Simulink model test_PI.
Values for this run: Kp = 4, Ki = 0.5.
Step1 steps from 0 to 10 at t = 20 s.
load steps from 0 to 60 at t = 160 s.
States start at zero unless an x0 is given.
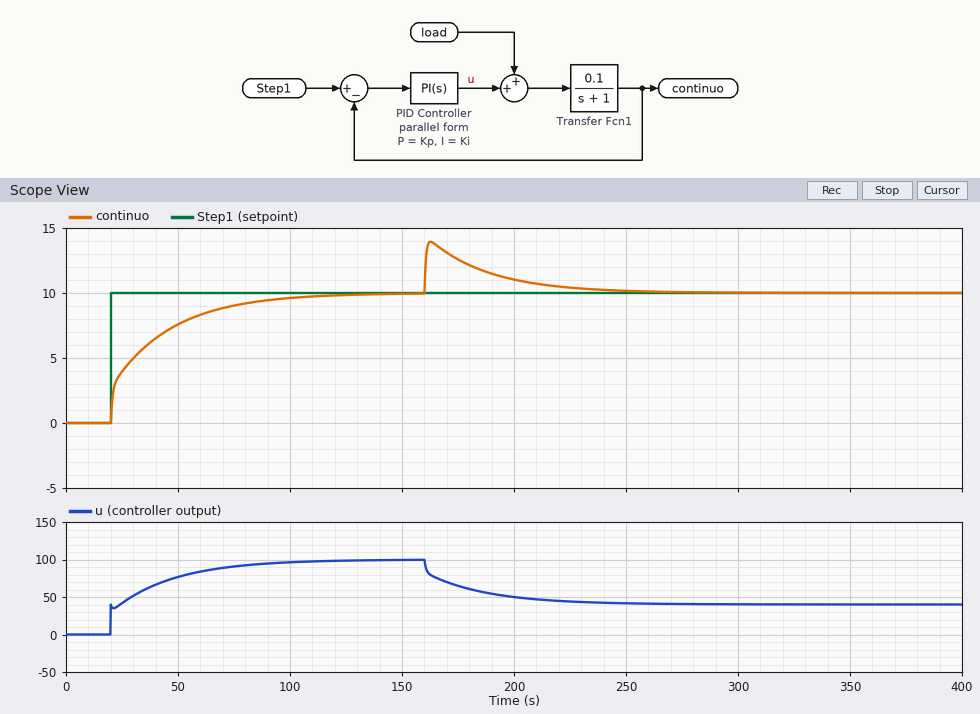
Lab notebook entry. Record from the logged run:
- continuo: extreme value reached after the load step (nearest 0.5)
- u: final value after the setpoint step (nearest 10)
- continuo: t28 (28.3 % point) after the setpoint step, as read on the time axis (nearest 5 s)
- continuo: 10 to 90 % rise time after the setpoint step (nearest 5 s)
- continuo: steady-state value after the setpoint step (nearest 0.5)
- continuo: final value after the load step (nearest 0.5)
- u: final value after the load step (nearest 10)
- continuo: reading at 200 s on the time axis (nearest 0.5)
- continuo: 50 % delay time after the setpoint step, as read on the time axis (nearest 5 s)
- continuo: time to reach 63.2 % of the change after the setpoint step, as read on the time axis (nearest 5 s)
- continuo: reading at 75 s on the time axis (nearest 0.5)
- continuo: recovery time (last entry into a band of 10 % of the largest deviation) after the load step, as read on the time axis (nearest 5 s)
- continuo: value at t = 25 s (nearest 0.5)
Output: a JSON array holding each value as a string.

["14.0", "100", "20 s", "55 s", "10.0", "10.0", "40", "11.0", "30 s", "40 s", "9.0", "225 s", "4.0"]
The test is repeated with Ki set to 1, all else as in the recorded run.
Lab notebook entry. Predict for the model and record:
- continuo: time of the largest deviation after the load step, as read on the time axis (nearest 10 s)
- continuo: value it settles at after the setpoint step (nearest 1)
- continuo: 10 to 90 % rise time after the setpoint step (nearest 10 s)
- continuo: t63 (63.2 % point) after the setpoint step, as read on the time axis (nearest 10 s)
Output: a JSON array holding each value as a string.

["160 s", "10", "30 s", "30 s"]
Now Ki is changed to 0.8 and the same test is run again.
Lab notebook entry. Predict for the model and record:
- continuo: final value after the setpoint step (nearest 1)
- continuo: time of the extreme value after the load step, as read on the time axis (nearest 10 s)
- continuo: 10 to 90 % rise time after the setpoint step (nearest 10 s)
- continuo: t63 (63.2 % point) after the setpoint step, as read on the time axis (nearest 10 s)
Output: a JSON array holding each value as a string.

["10", "160 s", "30 s", "30 s"]
